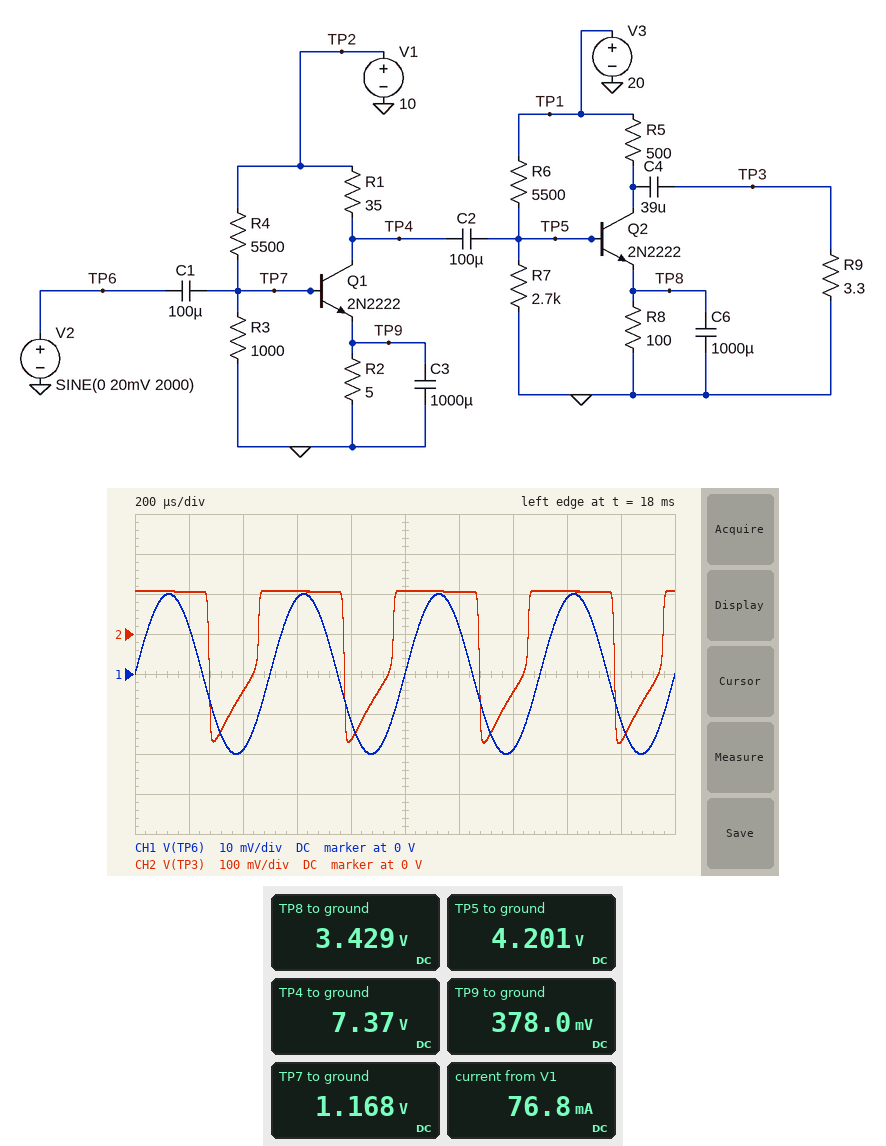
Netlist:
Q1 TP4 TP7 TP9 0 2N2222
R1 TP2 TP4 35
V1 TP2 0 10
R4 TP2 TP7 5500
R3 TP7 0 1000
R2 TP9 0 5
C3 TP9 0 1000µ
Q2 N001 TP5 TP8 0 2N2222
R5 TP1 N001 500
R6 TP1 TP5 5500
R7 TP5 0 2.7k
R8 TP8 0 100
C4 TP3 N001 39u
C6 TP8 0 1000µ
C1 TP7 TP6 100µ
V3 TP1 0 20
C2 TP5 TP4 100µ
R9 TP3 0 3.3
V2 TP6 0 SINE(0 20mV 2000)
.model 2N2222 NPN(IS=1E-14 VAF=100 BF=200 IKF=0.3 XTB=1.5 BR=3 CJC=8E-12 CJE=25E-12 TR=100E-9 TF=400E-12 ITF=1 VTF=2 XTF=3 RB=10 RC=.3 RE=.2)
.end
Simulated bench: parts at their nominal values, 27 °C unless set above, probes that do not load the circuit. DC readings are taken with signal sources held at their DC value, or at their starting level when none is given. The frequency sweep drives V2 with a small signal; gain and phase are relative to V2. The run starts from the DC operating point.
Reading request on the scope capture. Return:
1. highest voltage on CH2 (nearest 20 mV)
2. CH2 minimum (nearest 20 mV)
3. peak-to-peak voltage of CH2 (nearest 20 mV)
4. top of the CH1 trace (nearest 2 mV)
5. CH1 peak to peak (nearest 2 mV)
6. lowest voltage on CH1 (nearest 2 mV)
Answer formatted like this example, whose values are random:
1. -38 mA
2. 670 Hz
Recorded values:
1. 100 mV
2. -280 mV
3. 380 mV
4. 20 mV
5. 40 mV
6. -20 mV
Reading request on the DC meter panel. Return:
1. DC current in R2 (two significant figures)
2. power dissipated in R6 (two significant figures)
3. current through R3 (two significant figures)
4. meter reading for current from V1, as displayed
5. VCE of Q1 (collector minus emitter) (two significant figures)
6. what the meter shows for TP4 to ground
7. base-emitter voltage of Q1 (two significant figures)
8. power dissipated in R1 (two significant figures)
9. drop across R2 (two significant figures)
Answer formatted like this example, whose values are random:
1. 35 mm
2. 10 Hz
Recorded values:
1. 76 mA
2. 45 mW
3. 1.2 mA
4. 76.8 mA
5. 7.0 V
6. 7.37 V
7. 790 mV
8. 200 mW
9. 380 mV
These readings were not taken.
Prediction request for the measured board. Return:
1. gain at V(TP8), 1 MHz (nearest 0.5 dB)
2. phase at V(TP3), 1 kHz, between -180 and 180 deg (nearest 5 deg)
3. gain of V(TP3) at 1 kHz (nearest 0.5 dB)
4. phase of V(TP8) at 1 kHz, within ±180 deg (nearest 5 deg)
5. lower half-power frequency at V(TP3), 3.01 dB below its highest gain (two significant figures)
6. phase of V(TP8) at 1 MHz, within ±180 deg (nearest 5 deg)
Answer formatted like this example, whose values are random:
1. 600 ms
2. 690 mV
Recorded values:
1. -67.0 dB
2. 55 deg
3. 20.0 dB
4. 135 deg
5. 920 Hz
6. 45 deg
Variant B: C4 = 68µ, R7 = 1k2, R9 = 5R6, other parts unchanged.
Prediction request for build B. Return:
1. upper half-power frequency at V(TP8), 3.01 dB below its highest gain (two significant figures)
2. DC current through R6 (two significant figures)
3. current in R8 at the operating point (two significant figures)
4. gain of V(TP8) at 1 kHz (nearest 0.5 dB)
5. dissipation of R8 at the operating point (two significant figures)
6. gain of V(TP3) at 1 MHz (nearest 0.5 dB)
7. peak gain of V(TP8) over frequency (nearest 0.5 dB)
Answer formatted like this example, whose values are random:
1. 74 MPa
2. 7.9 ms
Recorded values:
1. 450 Hz
2. 3.0 mA
3. 27 mA
4. 14.0 dB
5. 73 mW
6. 45.0 dB
7. 22.5 dB
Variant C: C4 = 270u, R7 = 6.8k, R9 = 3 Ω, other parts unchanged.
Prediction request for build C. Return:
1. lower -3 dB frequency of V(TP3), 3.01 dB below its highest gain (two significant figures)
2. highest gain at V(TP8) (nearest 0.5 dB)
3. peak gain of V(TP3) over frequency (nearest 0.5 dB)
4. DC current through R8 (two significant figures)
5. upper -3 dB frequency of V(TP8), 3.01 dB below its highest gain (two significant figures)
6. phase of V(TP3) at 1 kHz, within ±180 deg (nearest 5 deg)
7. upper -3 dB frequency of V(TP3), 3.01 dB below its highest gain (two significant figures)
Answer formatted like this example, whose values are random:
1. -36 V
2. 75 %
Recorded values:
1. 360 Hz
2. 1.5 dB
3. 17.0 dB
4. 35 mA
5. 540 Hz
6. 25 deg
7. 600 kHz
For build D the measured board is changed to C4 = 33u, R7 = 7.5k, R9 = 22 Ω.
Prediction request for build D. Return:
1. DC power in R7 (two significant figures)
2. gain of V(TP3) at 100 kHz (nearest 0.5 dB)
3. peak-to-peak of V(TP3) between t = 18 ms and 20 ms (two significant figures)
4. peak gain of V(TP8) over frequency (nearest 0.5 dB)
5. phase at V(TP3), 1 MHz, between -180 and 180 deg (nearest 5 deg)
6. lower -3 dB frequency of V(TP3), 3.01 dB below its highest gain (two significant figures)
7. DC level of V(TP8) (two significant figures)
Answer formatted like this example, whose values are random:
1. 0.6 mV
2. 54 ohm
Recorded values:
1. 2.5 mW
2. 19.5 dB
3. 1.7 V
4. -4.5 dB
5. -75 deg
6. 390 Hz
7. 3.5 V
